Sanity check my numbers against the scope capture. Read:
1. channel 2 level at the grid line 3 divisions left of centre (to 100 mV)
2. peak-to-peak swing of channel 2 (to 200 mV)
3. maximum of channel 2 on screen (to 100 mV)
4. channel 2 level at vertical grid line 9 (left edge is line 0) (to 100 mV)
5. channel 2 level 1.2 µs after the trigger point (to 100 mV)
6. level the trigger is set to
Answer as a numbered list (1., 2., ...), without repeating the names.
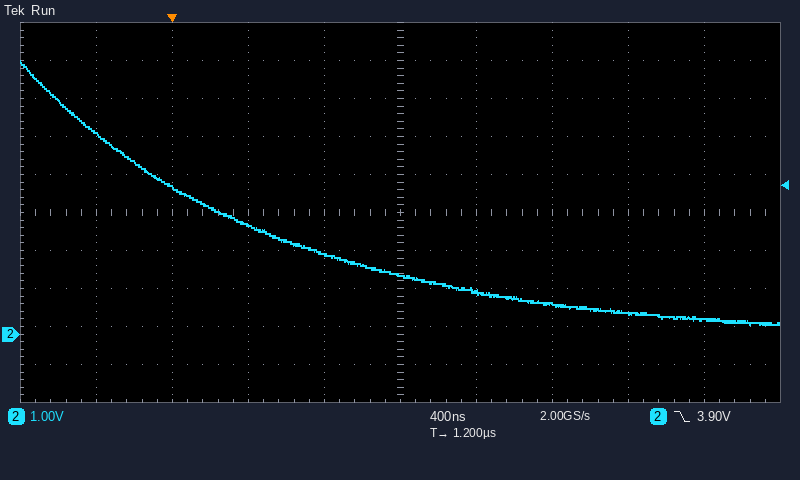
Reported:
1. 3.9 V
2. 7.0 V
3. 7.2 V
4. 400 mV
5. 1.5 V
6. 3.90 V
